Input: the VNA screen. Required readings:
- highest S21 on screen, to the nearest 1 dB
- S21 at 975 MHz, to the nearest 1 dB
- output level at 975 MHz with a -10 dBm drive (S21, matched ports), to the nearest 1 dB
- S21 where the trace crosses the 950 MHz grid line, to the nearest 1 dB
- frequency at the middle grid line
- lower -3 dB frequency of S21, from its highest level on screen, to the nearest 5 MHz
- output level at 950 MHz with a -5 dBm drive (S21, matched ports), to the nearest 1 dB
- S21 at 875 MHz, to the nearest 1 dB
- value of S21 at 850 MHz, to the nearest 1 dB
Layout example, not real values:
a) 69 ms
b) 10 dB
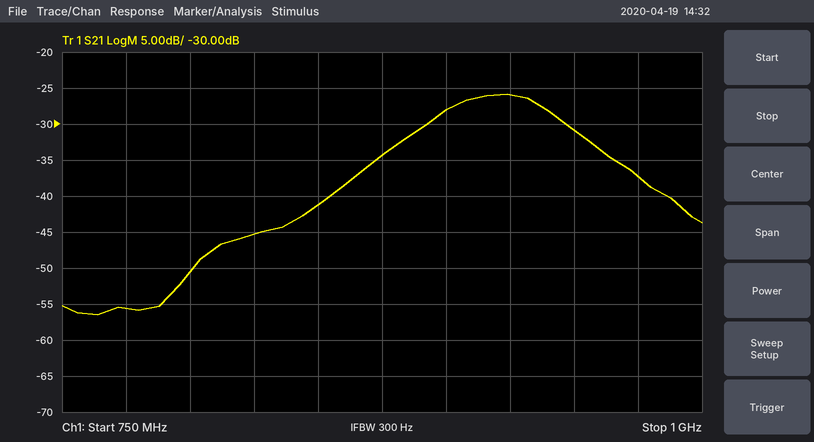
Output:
a) -26 dB
b) -37 dB
c) -47 dBm
d) -31 dB
e) 875 MHz
f) 895 MHz
g) -36 dBm
h) -34 dB
i) -41 dB
